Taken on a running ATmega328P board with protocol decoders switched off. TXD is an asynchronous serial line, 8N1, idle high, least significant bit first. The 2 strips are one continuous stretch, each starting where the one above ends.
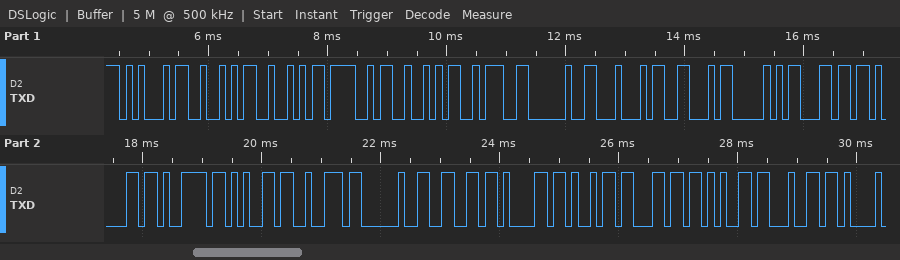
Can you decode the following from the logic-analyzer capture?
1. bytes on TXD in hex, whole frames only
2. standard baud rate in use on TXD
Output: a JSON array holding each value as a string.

["45 52 52 4F 52 3A 20 44 46 50 6C 61 79 65 72 20 66 61 69 6C 65 64", "9600 baud"]
